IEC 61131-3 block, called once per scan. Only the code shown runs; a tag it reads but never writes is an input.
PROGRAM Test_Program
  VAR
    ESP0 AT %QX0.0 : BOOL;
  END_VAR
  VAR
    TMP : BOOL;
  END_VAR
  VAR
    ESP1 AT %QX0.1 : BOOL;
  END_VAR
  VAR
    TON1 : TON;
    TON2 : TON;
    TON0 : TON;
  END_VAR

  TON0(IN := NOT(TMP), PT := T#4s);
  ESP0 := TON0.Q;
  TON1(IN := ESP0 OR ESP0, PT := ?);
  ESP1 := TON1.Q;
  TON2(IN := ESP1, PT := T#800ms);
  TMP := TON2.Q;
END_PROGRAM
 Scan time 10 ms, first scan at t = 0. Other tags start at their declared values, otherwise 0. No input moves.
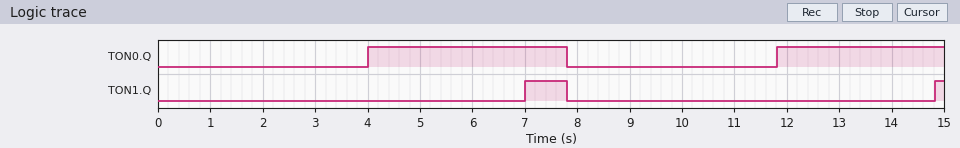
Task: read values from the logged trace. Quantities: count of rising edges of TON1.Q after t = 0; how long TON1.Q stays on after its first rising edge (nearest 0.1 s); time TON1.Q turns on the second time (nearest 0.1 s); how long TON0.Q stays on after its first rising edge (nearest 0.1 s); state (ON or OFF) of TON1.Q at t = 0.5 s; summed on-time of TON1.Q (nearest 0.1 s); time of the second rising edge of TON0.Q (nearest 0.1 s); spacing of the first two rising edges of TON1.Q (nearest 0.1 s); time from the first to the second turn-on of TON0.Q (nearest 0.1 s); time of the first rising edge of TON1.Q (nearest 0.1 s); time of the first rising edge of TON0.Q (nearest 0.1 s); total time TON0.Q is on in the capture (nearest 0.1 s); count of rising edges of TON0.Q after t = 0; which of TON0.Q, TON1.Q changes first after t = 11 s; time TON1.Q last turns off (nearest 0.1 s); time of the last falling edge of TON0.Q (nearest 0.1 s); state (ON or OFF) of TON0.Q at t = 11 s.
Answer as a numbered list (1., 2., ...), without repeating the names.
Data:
1. 2
2. 0.8 s
3. 14.8 s
4. 3.8 s
5. OFF
6. 1.0 s
7. 11.8 s
8. 7.8 s
9. 7.8 s
10. 7.0 s
11. 4.0 s
12. 7.0 s
13. 2
14. TON0.Q
15. 7.8 s
16. 7.8 s
17. OFF
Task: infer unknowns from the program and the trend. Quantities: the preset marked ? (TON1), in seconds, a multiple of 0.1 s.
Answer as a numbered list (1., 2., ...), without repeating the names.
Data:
1. 3.0 s
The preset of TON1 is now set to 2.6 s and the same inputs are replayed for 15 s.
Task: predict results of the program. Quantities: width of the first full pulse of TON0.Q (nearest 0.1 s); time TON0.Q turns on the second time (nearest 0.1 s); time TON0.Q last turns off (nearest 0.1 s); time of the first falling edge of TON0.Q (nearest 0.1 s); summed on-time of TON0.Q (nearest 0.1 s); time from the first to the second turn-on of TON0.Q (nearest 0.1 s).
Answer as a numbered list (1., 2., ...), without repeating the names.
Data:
1. 3.4 s
2. 11.4 s
3. 14.8 s
4. 7.4 s
5. 6.8 s
6. 7.4 s
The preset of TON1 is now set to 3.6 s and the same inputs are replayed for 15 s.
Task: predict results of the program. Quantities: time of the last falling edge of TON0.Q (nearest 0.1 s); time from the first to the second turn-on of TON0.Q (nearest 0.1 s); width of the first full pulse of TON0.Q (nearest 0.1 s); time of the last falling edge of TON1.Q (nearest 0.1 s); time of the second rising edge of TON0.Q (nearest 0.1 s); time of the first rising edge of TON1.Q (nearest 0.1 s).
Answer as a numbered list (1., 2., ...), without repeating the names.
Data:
1. 8.4 s
2. 8.4 s
3. 4.4 s
4. 8.4 s
5. 12.4 s
6. 7.6 s
